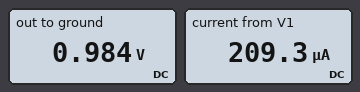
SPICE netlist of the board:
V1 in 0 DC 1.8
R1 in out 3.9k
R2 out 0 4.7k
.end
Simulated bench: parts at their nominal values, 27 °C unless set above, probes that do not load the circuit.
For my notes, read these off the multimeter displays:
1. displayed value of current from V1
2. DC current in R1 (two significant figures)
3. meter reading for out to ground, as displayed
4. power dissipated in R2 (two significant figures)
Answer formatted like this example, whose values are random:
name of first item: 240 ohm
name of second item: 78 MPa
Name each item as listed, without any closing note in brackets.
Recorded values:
displayed value of current from V1: 209.3 µA
DC current in R1: 210 µA
meter reading for out to ground, as displayed: 0.984 V
power dissipated in R2: 210 µW
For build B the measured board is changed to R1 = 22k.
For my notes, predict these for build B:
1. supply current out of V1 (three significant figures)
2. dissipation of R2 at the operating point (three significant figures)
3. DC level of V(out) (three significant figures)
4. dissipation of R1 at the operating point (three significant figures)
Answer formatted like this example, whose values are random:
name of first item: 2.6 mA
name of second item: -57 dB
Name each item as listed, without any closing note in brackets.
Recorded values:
supply current out of V1: 67.4 µA
dissipation of R2 at the operating point: 21.4 µW
DC level of V(out): 317 mV
dissipation of R1 at the operating point: 100 µW
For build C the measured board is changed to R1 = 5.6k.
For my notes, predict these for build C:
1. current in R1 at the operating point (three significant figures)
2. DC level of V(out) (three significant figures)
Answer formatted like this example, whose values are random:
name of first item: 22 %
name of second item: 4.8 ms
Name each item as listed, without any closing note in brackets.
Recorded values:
current in R1 at the operating point: 175 µA
DC level of V(out): 821 mV
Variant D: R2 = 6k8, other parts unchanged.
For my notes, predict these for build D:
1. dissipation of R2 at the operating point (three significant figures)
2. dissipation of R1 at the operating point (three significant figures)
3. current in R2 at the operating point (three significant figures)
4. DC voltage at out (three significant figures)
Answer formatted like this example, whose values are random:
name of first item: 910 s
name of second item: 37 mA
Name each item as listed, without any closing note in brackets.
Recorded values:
dissipation of R2 at the operating point: 192 µW
dissipation of R1 at the operating point: 110 µW
current in R2 at the operating point: 168 µA
DC voltage at out: 1.14 V
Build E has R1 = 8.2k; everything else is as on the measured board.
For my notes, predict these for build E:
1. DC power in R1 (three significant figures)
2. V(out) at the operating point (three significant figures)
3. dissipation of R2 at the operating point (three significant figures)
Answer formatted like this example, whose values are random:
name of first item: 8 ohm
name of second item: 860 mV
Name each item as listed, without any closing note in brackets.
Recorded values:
DC power in R1: 160 µW
V(out) at the operating point: 656 mV
dissipation of R2 at the operating point: 91.5 µW
